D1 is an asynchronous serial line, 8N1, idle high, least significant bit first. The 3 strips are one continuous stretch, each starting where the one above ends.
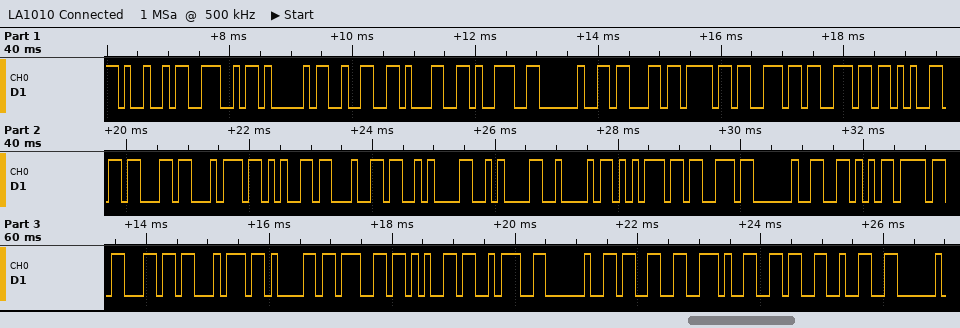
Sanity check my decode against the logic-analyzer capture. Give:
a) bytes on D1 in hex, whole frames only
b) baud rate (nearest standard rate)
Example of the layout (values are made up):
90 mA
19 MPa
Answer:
0x49 0x4E 0x41 0x32 0x31 0x39 0x20 0x63 0x6F 0x6E 0x6E 0x65 0x63 0x74 0x65 0x64 0x0A 0x0A 0x42 0x75 0x73 0x20 0x56 0x6F 0x6C 0x74 0x61 0x67 0x65 0x3A 0x20 0x33 0x2E 0x36 0x32
9600 baud
